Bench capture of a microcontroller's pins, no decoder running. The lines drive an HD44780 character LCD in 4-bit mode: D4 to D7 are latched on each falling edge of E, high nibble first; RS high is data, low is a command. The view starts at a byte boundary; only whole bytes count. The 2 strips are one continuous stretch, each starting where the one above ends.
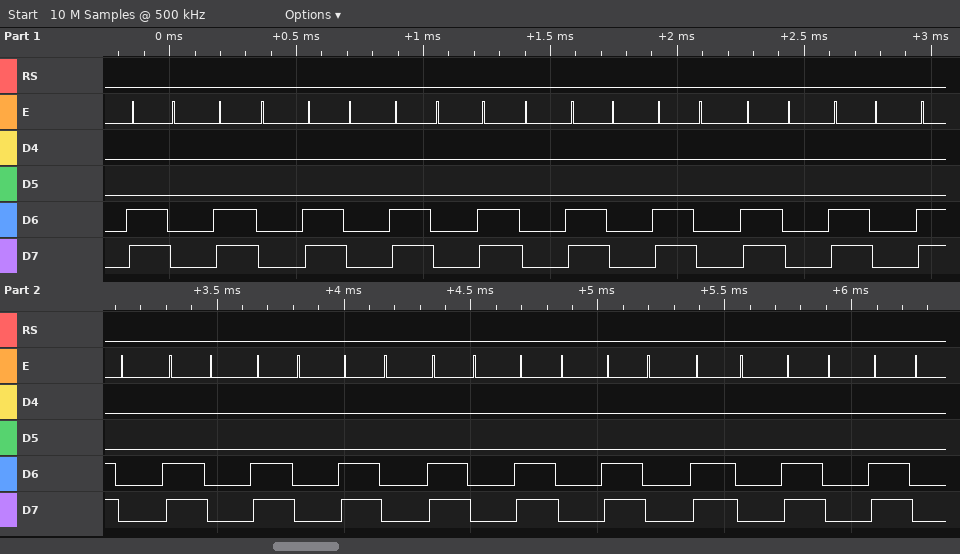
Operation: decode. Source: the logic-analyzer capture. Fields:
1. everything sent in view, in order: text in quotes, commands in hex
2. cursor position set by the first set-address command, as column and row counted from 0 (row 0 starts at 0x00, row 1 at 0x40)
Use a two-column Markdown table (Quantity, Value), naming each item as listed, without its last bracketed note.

| Quantity | Value |
|---|---|
| everything sent in view, in order: text in quotes, commands in hex | 0xC0 0xC0 0xC0 0xC0 0xC0 0xC0 0xC0 0xC0 0xC0 0xC0 0xC0 0xC0 0xC0 0xC0 0xC0 0xC0 0xC0 0xC0 0xC0 |
| cursor position set by the first set-address command, as column and row counted from 0 | column 0, row 1 |
